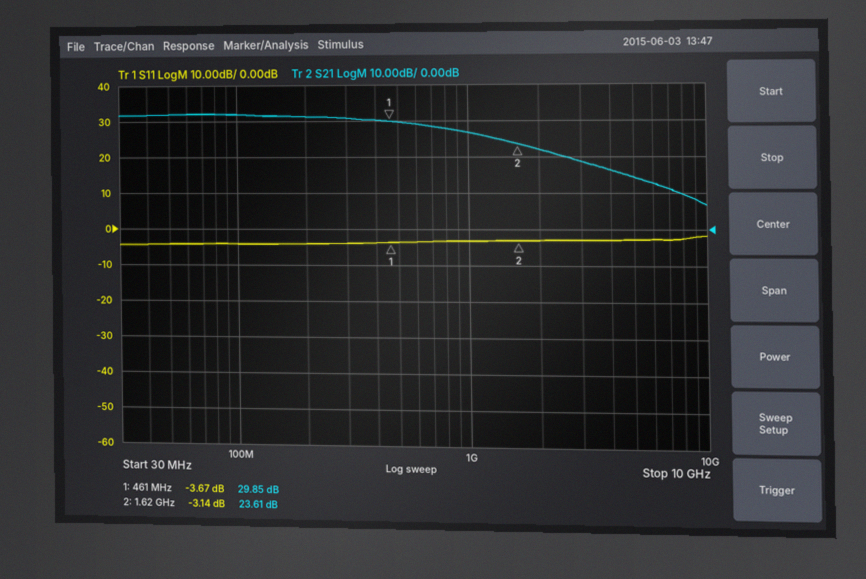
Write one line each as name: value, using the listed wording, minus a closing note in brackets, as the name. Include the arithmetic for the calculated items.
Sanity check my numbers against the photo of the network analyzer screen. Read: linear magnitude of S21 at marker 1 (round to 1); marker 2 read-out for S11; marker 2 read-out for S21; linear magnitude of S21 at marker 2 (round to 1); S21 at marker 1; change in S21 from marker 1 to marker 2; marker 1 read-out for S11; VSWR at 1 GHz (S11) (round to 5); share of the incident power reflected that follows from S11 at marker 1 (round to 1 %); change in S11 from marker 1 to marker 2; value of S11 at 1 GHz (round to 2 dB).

linear magnitude of S21 at marker 1: 10^(29.85/20) ≈ 31
marker 2 read-out for S11: -3.14 dB
marker 2 read-out for S21: 23.61 dB
linear magnitude of S21 at marker 2: 10^(23.61/20) ≈ 15
S21 at marker 1: 29.85 dB
change in S21 from marker 1 to marker 2: 23.61 − (29.85) = -6.24 dB
marker 1 read-out for S11: -3.67 dB
VSWR at 1 GHz (S11): |Γ| = 10^(-4/20) = 0.6310; VSWR = (1 + 0.6310)/(1 − 0.6310) ≈ 4.42, so 5 to the nearest 5
share of the incident power reflected that follows from S11 at marker 1: 10^(-3.67/10) ≈ 43 %
change in S11 from marker 1 to marker 2: -3.14 − (-3.67) = 0.53 dB
value of S11 at 1 GHz: -4 dB
